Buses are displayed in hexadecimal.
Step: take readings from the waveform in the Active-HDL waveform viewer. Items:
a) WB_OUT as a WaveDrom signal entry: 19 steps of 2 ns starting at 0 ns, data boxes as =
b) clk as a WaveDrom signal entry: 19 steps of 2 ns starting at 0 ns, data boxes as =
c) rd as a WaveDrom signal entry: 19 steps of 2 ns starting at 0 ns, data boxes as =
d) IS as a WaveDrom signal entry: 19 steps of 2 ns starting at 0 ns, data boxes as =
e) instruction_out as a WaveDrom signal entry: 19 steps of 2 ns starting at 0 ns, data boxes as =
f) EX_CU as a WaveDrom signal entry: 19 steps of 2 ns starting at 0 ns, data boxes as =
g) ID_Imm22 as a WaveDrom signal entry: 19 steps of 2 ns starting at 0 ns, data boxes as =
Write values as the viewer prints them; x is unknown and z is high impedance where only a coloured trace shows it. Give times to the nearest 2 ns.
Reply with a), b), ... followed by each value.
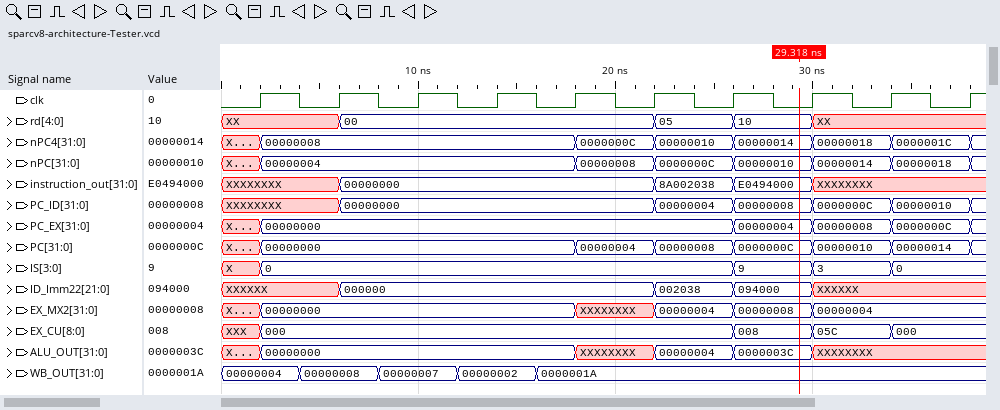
a) {name: 'WB_OUT', wave: '=.=.=.=.=..........', data: '00000004 00000008 00000007 00000002 0000001A'}
b) {name: 'clk', wave: '0101010101010101010'}
c) {name: 'rd', wave: 'x..=.......=.=.x...', data: '00 05 10'}
d) {name: 'IS', wave: 'x=...........=.=.=.', data: '0 9 3 0'}
e) {name: 'instruction_out', wave: 'x..=.......=.=.x...', data: '00000000 8A002038 E0494000'}
f) {name: 'EX_CU', wave: 'x=...........=.=.=.', data: '000 008 05C 000'}
g) {name: 'ID_Imm22', wave: 'x..=.......=.=.x...', data: '000000 002038 094000'}
